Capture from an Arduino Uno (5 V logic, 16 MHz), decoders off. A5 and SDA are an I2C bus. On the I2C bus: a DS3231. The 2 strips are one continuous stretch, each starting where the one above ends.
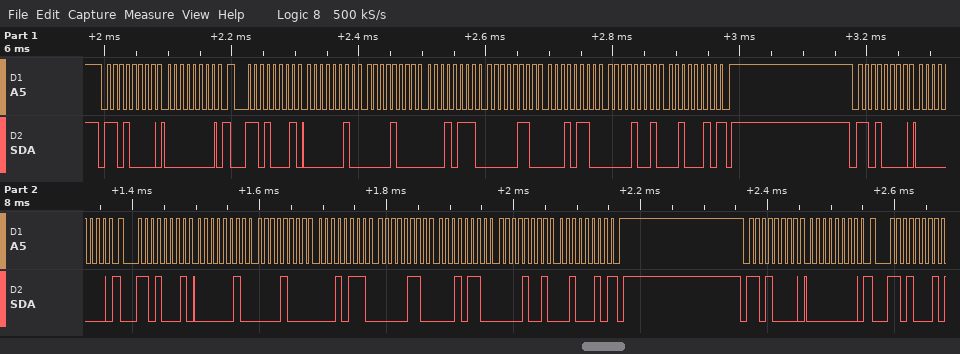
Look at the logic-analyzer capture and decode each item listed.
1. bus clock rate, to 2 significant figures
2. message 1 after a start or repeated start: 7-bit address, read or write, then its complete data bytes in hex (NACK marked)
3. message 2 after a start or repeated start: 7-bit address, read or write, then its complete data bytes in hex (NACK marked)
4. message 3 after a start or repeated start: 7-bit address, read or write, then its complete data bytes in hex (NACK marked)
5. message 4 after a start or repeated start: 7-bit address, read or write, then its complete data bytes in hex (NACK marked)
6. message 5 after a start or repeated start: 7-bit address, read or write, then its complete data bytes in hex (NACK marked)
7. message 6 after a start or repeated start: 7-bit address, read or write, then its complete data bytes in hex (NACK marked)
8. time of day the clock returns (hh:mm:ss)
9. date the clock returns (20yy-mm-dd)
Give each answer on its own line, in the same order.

100 kHz
0x68 write: 00
0x68 read: 02 08 17 06 16 09 22 NACK
0x68 write: 00
0x68 read: 02 08 17 06 16 09 22 NACK
0x68 write: 00
0x68 read
17:08:02
2022-09-16
